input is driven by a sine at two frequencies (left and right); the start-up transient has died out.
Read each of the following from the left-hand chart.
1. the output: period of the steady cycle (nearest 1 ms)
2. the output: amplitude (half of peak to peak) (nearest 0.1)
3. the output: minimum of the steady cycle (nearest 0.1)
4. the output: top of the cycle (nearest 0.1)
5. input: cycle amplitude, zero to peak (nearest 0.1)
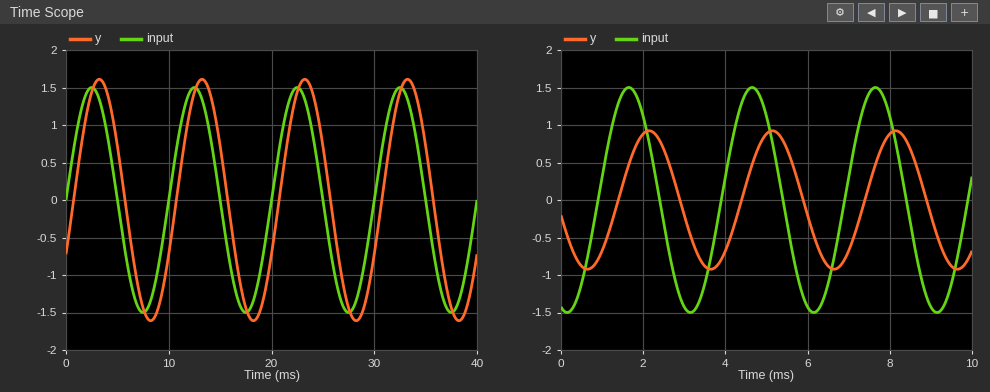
10 ms
1.6
-1.6
1.6
1.5
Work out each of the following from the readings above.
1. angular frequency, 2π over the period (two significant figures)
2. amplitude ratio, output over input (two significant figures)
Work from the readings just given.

0.63 rad/ms
1.1
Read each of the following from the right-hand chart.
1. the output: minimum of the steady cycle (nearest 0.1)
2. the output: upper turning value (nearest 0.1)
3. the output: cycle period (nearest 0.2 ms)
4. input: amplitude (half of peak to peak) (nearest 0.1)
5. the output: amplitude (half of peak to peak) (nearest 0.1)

-0.9
0.9
3.0 ms
1.5
0.9
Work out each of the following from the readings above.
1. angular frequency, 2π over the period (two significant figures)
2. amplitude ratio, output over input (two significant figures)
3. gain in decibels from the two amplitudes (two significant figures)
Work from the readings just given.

2.1 rad/ms
0.60
-4.4 dB
